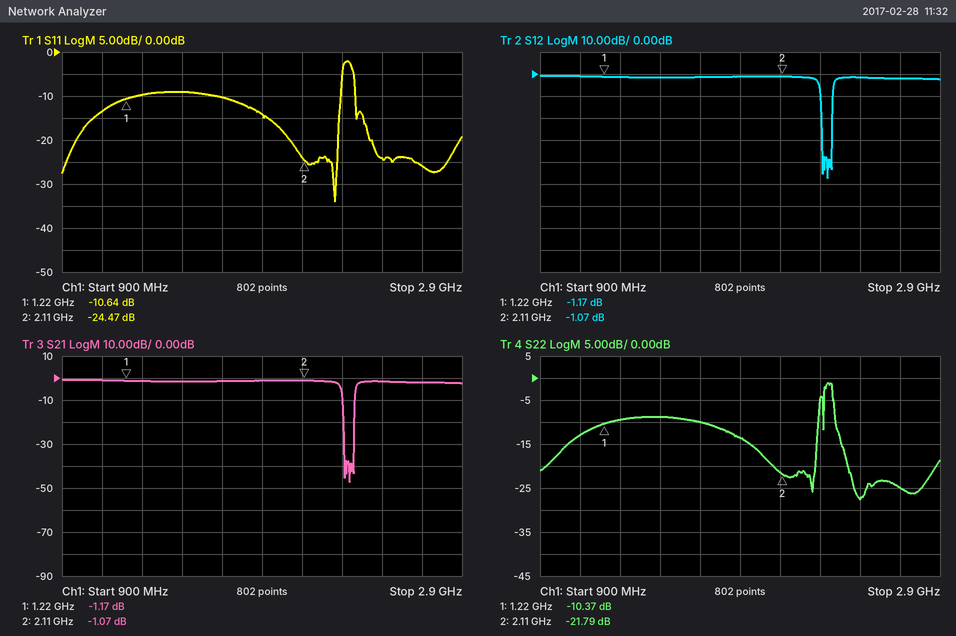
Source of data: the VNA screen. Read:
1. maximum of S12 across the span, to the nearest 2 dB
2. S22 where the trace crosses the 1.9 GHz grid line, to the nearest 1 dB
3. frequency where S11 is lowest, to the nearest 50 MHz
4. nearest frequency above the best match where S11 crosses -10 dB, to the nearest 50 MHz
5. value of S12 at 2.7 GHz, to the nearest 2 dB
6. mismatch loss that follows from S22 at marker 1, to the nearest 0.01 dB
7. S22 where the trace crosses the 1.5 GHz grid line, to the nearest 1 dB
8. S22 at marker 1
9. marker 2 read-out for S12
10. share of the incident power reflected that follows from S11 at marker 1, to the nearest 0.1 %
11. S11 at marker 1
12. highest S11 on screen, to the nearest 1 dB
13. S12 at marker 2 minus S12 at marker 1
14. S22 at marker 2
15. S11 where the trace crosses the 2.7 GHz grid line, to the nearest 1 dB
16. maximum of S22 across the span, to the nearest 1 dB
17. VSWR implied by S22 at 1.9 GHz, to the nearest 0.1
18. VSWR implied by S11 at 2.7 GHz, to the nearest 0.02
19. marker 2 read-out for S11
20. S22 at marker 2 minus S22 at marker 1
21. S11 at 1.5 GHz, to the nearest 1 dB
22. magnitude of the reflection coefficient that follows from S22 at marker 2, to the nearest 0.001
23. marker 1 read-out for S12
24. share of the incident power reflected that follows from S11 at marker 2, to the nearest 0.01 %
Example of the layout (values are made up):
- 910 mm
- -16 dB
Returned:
- 0 dB
- -14 dB
- 2.25 GHz
- 2.30 GHz
- -2 dB
- 0.42 dB
- -9 dB
- -10.37 dB
- -1.07 dB
- 8.6 %
- -10.64 dB
- -2 dB
- 0.10 dB
- -21.79 dB
- -26 dB
- -1 dB
- 1.5
- 1.10
- -24.47 dB
- -11.42 dB
- -9 dB
- 0.081
- -1.17 dB
- 0.36 %
